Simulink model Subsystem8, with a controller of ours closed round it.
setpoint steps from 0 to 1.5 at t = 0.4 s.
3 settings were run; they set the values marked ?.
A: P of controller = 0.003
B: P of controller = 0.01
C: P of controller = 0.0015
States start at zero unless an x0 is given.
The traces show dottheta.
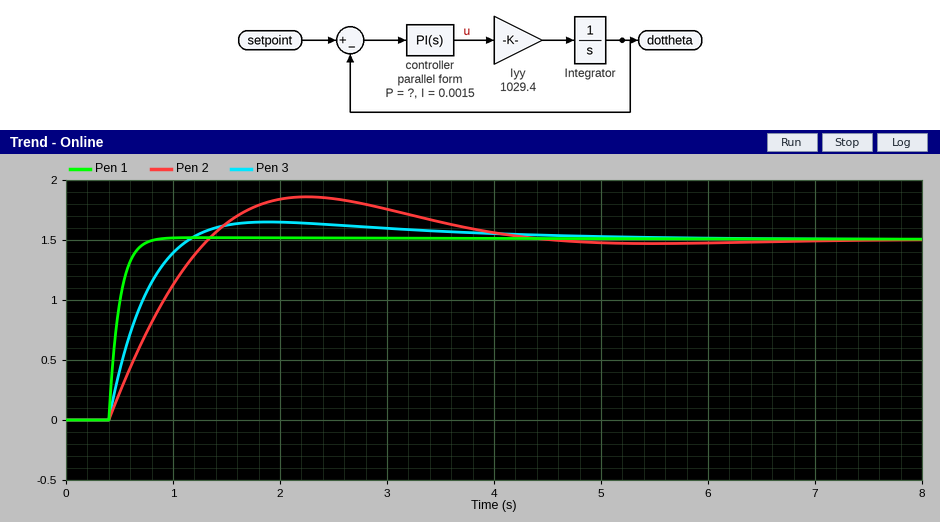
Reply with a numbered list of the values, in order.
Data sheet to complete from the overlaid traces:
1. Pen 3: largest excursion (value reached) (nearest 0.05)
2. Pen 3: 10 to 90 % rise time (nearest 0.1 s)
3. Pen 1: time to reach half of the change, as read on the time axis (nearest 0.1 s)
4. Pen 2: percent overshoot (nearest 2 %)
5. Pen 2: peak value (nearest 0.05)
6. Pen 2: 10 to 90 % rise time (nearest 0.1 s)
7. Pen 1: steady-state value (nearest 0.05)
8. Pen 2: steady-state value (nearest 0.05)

1. 1.65
2. 0.5 s
3. 0.5 s
4. 24 %
5. 1.85
6. 0.7 s
7. 1.50
8. 1.50
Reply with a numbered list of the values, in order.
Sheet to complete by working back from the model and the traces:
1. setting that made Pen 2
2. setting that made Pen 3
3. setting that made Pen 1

1. C
2. A
3. B
